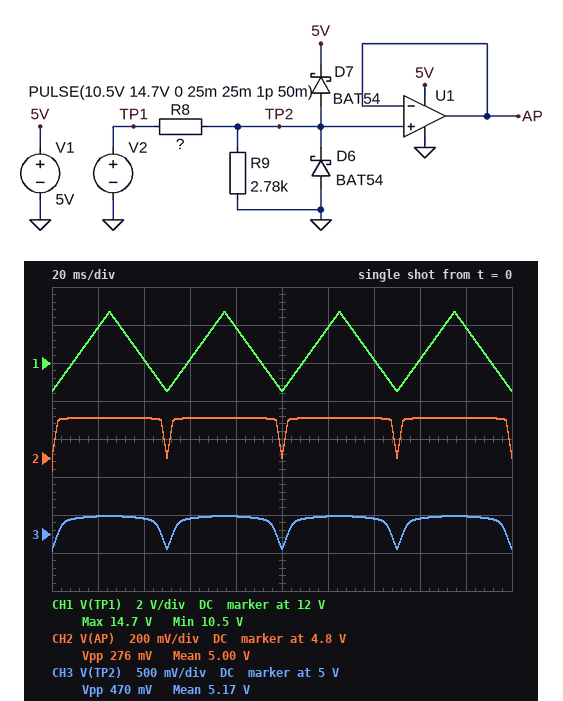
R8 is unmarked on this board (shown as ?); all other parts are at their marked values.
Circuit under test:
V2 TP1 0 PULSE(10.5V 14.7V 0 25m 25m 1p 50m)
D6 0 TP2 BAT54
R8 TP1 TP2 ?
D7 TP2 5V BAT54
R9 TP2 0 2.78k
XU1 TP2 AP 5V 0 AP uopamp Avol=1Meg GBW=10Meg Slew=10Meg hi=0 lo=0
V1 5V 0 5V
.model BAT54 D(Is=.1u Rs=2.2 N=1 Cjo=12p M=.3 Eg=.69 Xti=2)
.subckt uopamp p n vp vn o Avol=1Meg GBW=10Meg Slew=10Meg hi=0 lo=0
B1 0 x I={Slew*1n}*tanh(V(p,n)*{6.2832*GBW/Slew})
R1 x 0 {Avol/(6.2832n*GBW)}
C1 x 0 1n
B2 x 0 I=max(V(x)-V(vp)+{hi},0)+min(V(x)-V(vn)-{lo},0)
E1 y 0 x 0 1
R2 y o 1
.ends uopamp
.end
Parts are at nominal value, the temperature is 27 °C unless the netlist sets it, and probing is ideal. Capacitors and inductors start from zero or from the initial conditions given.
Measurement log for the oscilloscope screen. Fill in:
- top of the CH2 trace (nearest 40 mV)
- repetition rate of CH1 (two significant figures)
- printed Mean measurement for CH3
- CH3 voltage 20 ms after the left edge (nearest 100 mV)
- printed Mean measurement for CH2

5.00 V
20 Hz
5.17 V
5.2 V
5.00 V
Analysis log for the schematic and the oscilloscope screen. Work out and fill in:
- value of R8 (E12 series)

3.3 kΩ
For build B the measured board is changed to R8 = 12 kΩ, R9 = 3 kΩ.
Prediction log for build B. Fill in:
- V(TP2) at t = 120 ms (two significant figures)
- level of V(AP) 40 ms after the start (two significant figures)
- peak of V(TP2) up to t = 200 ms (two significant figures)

2.8 V
2.4 V
2.9 V
